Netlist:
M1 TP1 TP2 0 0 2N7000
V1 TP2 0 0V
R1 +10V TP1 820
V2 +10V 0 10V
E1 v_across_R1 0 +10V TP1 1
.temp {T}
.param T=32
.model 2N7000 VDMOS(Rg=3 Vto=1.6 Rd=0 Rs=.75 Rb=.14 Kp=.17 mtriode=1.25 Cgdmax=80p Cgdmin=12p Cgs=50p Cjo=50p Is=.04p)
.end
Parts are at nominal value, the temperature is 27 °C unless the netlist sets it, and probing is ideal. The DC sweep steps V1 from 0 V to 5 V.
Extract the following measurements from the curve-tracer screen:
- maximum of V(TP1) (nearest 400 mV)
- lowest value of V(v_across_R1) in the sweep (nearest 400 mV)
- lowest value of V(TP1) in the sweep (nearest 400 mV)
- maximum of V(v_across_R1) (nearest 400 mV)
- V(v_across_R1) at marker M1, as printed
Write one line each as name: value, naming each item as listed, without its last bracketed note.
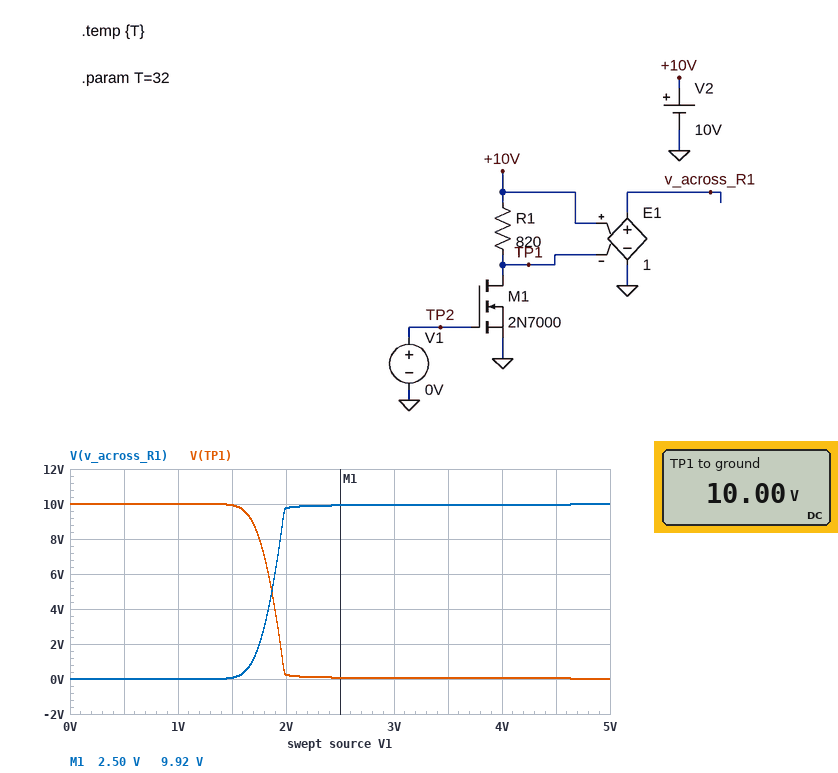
maximum of V(TP1): 10.0 V
lowest value of V(v_across_R1) in the sweep: 0 V
lowest value of V(TP1) in the sweep: 0 V
maximum of V(v_across_R1): 10.0 V
V(v_across_R1) at marker M1, as printed: 9.92 V
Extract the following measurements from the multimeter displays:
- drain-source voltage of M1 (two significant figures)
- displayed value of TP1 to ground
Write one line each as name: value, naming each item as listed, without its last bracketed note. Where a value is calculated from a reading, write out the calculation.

drain-source voltage of M1: 10 V = 10 V
displayed value of TP1 to ground: 10.00 V
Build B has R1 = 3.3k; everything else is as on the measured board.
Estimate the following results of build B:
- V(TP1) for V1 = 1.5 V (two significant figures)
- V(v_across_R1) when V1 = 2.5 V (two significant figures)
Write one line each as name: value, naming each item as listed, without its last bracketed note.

V(TP1) for V1 = 1.5 V: 9.7 V
V(v_across_R1) when V1 = 2.5 V: 10 V
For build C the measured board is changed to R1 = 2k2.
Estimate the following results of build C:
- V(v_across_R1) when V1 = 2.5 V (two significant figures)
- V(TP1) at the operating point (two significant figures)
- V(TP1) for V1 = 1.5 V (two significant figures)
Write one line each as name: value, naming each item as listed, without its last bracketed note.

V(v_across_R1) when V1 = 2.5 V: 10 V
V(TP1) at the operating point: 10 V
V(TP1) for V1 = 1.5 V: 9.8 V
